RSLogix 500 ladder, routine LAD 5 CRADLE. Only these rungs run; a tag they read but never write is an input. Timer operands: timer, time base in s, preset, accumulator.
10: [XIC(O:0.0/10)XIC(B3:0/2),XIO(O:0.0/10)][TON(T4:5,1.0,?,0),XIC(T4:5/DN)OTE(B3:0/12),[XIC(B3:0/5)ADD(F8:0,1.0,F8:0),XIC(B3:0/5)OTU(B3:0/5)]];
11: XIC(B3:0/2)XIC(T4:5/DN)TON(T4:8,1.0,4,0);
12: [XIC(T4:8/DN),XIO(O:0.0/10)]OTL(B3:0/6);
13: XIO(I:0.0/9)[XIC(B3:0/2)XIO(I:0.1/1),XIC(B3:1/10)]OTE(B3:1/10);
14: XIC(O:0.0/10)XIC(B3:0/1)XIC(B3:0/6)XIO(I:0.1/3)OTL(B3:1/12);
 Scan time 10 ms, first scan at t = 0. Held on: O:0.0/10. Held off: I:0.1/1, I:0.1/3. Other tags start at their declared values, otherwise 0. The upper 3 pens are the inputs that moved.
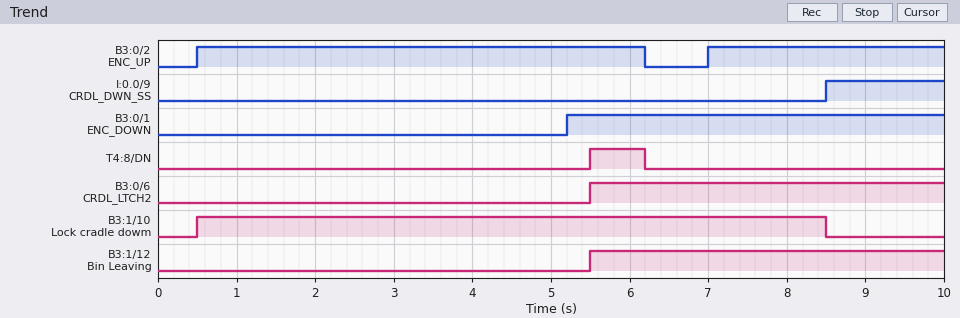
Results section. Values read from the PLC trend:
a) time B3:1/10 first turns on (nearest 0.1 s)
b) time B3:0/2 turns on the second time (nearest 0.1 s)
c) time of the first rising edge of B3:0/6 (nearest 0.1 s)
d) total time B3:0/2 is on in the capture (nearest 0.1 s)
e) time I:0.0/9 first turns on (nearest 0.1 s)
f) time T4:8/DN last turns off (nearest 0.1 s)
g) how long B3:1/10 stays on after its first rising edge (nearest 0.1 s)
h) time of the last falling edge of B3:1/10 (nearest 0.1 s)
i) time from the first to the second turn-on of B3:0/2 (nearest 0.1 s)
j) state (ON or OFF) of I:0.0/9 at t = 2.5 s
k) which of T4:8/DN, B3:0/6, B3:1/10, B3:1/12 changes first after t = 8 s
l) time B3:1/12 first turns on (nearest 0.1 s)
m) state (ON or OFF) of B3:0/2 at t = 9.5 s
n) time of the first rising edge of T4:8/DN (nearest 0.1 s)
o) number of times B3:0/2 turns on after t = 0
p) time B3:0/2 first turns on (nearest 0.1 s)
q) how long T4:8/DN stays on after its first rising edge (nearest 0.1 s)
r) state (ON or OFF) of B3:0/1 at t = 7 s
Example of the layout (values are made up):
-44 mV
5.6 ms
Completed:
0.5 s
7.0 s
5.5 s
8.7 s
8.5 s
6.2 s
8.0 s
8.5 s
6.5 s
OFF
B3:1/10
5.5 s
ON
5.5 s
2
0.5 s
0.7 s
ON
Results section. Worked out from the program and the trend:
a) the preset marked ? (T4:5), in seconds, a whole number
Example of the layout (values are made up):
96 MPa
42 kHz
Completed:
1 s
